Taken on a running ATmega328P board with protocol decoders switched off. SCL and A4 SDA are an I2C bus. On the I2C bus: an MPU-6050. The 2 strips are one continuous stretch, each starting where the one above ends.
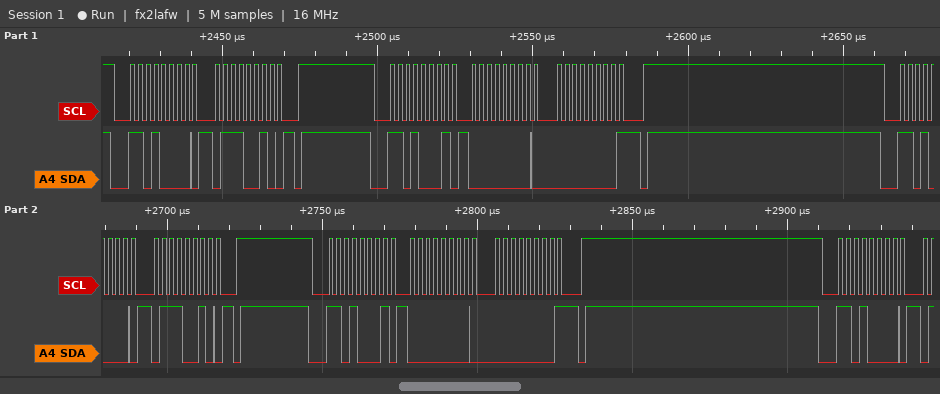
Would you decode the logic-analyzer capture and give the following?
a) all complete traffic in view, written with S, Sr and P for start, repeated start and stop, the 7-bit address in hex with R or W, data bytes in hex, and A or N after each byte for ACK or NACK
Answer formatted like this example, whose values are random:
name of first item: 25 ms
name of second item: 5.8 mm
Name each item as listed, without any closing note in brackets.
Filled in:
all complete traffic in view, written with S, Sr and P for start, repeated start and stop, the 7-bit address in hex with R or W, data bytes in hex, and A or N after each byte for ACK or NACK: S 68W A 72 A P S 68R A 00 A 00 N P S 68W A 72 A P S 68R A 00 A 00 N P S 68W A
